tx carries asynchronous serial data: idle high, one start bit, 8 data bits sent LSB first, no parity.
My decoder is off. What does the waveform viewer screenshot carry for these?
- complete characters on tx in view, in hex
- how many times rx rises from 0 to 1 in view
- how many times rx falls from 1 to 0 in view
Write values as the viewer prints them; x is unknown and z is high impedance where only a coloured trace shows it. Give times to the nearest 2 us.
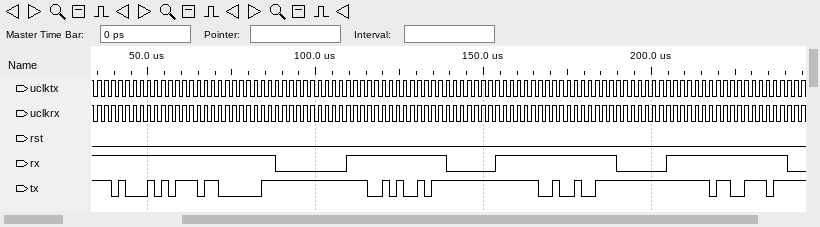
51, 03, 4A, 92, 73
3
4
